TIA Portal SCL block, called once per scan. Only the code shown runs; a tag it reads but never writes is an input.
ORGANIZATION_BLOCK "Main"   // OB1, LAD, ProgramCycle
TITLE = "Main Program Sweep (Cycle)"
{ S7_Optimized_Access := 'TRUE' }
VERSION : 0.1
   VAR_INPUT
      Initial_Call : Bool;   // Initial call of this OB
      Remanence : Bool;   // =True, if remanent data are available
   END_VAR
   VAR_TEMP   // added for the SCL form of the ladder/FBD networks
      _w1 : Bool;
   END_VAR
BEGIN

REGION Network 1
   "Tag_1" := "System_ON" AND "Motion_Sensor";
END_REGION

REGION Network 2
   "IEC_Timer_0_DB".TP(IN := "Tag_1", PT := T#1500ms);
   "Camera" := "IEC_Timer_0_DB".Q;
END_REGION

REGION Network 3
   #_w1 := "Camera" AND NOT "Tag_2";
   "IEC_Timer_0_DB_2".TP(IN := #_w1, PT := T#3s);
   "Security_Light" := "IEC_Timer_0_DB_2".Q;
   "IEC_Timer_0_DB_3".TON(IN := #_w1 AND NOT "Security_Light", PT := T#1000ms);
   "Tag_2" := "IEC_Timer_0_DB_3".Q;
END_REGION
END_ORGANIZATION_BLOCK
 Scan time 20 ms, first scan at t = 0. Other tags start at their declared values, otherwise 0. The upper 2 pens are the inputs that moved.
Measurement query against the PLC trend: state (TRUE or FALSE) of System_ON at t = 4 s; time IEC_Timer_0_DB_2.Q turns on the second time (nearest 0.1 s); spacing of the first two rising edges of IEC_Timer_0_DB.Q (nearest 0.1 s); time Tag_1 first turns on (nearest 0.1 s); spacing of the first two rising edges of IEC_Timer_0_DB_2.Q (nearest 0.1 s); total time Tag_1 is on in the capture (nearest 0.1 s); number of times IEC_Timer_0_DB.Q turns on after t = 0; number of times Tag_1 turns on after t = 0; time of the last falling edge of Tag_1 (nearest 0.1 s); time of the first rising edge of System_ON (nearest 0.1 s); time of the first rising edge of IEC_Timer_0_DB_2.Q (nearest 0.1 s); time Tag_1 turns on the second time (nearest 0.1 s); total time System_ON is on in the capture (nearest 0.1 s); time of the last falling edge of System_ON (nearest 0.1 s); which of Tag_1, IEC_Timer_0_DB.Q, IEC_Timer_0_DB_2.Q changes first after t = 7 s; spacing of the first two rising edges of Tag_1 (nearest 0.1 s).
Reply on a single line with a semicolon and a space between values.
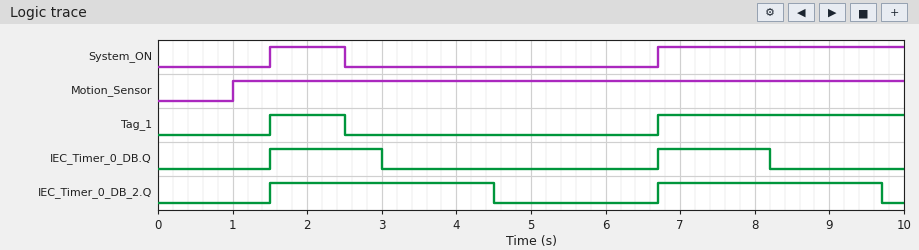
FALSE; 6.7 s; 5.2 s; 1.5 s; 5.2 s; 4.3 s; 2; 2; 2.5 s; 1.5 s; 1.5 s; 6.7 s; 4.3 s; 2.5 s; IEC_Timer_0_DB.Q; 5.2 s
